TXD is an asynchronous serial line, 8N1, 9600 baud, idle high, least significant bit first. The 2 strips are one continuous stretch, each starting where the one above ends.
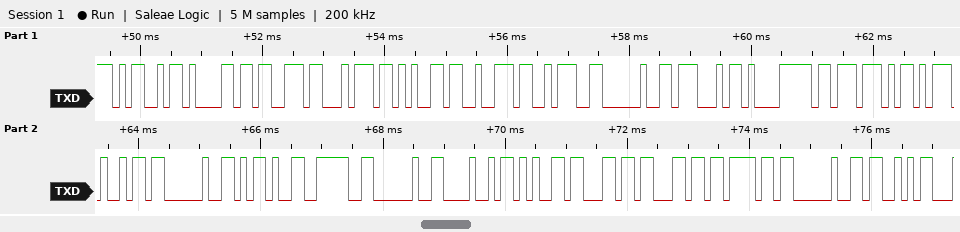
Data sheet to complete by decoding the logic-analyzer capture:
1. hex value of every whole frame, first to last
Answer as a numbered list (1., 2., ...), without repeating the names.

1. 0x4D 0x61 0x73 0x74 0x65 0x72 0x3A 0x20 0x47 0xE1 0xBB 0xAD 0x69 0x20 0x2D 0x3E 0x20 0x48 0x65 0x6C 0x6C 0x6F 0x20 0x53
